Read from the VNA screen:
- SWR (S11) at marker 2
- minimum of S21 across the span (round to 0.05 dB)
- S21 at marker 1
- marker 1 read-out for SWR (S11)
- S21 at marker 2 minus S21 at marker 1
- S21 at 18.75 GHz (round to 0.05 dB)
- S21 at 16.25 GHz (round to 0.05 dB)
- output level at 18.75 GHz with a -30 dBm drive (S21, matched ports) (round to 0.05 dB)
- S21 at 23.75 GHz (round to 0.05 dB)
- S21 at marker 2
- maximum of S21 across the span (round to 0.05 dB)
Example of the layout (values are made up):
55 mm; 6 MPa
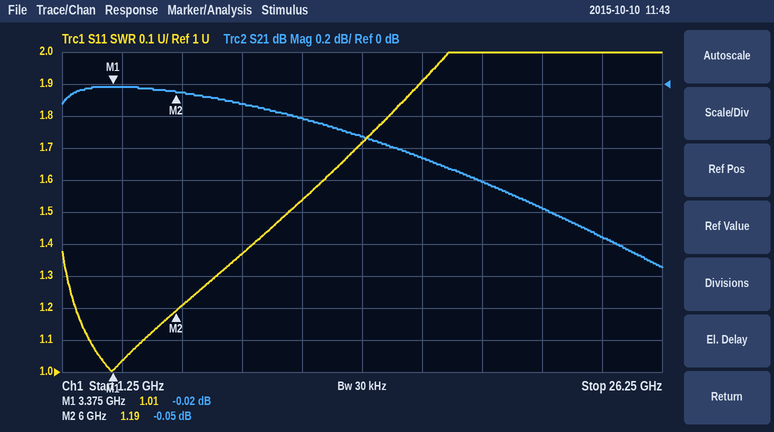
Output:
1.19; -1.15 dB; -0.02 dB; 1.01; -0.03 dB; -0.60 dB; -0.45 dB; -30.60 dBm; -0.95 dB; -0.05 dB; 0.00 dB
